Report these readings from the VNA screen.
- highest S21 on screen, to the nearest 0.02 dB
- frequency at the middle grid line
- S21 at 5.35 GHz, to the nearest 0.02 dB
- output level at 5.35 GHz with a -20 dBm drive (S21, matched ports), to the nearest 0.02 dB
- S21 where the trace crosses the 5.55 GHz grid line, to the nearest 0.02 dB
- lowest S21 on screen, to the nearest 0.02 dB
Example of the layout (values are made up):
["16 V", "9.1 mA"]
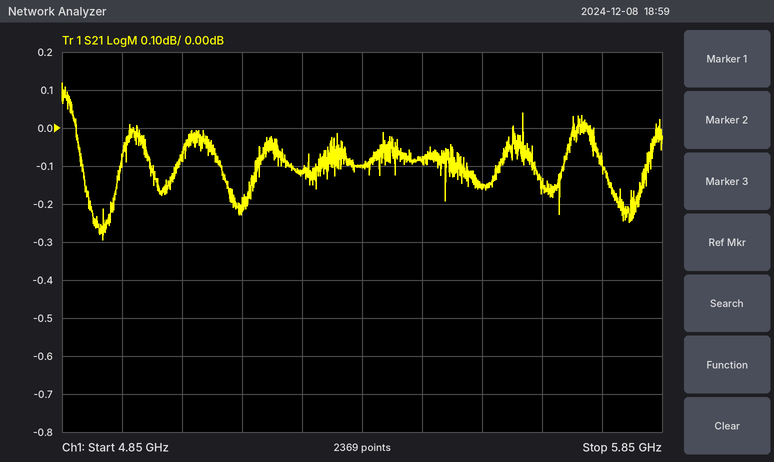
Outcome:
["0.12 dB", "5.35 GHz", "-0.10 dB", "-20.10 dBm", "-0.16 dB", "-0.30 dB"]
